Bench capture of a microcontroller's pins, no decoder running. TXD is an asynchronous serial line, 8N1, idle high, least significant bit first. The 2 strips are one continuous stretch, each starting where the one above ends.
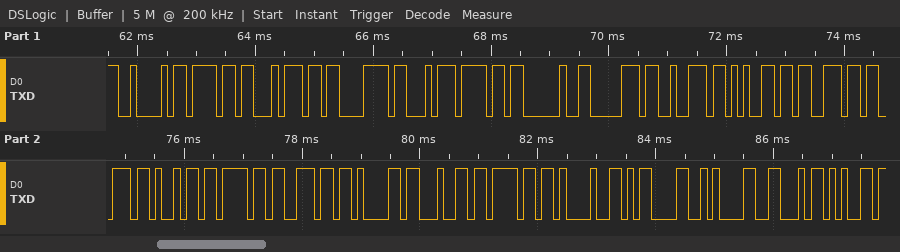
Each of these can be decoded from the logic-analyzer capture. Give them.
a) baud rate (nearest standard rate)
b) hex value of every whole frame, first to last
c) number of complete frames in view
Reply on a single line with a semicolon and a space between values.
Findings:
9600 baud; 42 6F 74 C3 A3 6F 20 70 72 65 73 73 69 6F 6E 61 64 6F 21 0D 0A 46 65; 23
